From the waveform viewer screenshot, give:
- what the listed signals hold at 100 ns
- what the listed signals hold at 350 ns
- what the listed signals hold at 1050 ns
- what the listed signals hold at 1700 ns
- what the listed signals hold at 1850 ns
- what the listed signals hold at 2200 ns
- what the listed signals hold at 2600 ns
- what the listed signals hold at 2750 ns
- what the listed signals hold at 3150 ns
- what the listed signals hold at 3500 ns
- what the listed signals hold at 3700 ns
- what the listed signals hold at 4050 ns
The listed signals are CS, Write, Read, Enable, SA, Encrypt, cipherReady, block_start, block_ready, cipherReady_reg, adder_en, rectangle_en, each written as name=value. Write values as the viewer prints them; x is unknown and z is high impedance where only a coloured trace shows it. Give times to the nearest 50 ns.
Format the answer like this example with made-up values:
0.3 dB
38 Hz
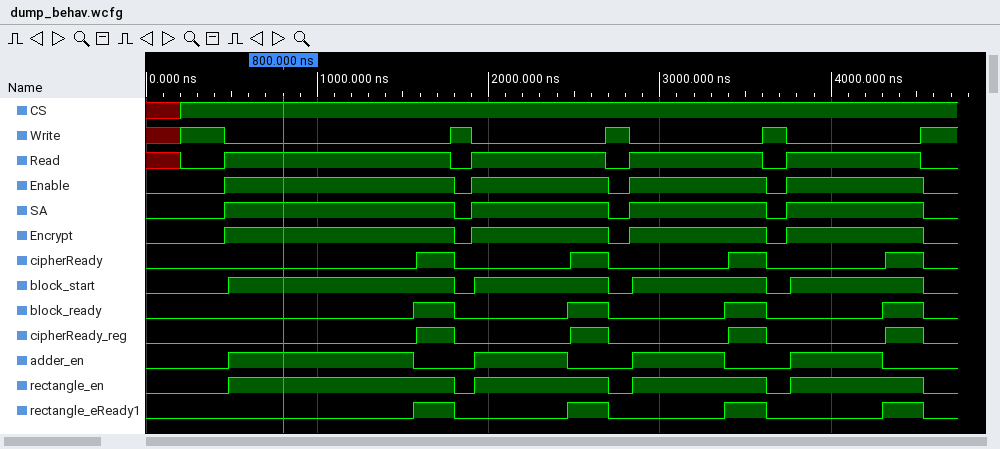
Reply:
CS=x, Write=x, Read=x, Enable=0, SA=0, Encrypt=0, cipherReady=0, block_start=0, block_ready=0, cipherReady_reg=0, adder_en=0, rectangle_en=0
CS=1, Write=1, Read=0, Enable=0, SA=0, Encrypt=0, cipherReady=0, block_start=0, block_ready=0, cipherReady_reg=0, adder_en=0, rectangle_en=0
CS=1, Write=0, Read=1, Enable=1, SA=1, Encrypt=1, cipherReady=0, block_start=1, block_ready=0, cipherReady_reg=0, adder_en=1, rectangle_en=1
CS=1, Write=0, Read=1, Enable=1, SA=1, Encrypt=1, cipherReady=1, block_start=1, block_ready=1, cipherReady_reg=1, adder_en=0, rectangle_en=1
CS=1, Write=1, Read=0, Enable=0, SA=0, Encrypt=0, cipherReady=0, block_start=0, block_ready=0, cipherReady_reg=0, adder_en=0, rectangle_en=0
CS=1, Write=0, Read=1, Enable=1, SA=1, Encrypt=1, cipherReady=0, block_start=1, block_ready=0, cipherReady_reg=0, adder_en=1, rectangle_en=1
CS=1, Write=0, Read=1, Enable=1, SA=1, Encrypt=1, cipherReady=1, block_start=1, block_ready=1, cipherReady_reg=1, adder_en=0, rectangle_en=1
CS=1, Write=1, Read=0, Enable=0, SA=0, Encrypt=0, cipherReady=0, block_start=0, block_ready=0, cipherReady_reg=0, adder_en=0, rectangle_en=0
CS=1, Write=0, Read=1, Enable=1, SA=1, Encrypt=1, cipherReady=0, block_start=1, block_ready=0, cipherReady_reg=0, adder_en=1, rectangle_en=1
CS=1, Write=0, Read=1, Enable=1, SA=1, Encrypt=1, cipherReady=1, block_start=1, block_ready=1, cipherReady_reg=1, adder_en=0, rectangle_en=1
CS=1, Write=1, Read=0, Enable=0, SA=0, Encrypt=0, cipherReady=0, block_start=0, block_ready=0, cipherReady_reg=0, adder_en=0, rectangle_en=0
CS=1, Write=0, Read=1, Enable=1, SA=1, Encrypt=1, cipherReady=0, block_start=1, block_ready=0, cipherReady_reg=0, adder_en=1, rectangle_en=1
